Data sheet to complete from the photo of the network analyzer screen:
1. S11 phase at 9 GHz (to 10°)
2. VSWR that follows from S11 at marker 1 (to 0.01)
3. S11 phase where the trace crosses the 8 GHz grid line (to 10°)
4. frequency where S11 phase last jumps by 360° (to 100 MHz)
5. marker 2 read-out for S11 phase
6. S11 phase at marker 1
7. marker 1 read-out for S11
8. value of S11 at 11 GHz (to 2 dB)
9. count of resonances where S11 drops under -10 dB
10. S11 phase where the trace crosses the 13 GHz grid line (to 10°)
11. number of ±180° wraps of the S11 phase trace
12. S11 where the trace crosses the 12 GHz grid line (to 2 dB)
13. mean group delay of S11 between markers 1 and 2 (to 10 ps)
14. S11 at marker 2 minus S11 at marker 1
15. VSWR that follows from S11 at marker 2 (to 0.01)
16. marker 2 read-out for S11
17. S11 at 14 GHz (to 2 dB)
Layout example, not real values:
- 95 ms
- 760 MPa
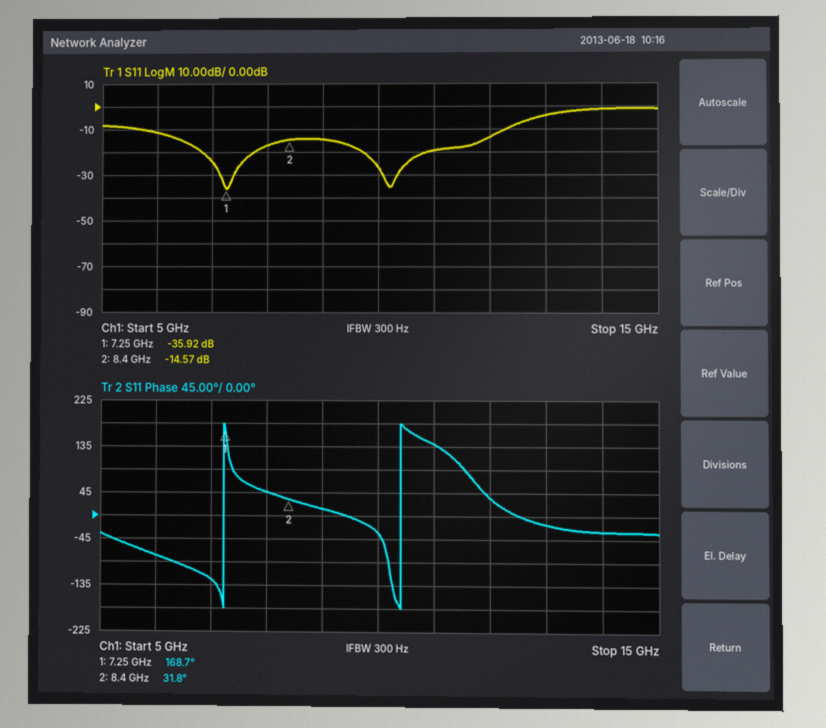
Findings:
- 10°
- 1.03
- 50°
- 10.4 GHz
- 31.8°
- 168.7°
- -35.92 dB
- -20 dB
- 2
- -20°
- 2
- -14 dB
- 330 ps
- 21.35 dB
- 1.46
- -14.57 dB
- -2 dB
